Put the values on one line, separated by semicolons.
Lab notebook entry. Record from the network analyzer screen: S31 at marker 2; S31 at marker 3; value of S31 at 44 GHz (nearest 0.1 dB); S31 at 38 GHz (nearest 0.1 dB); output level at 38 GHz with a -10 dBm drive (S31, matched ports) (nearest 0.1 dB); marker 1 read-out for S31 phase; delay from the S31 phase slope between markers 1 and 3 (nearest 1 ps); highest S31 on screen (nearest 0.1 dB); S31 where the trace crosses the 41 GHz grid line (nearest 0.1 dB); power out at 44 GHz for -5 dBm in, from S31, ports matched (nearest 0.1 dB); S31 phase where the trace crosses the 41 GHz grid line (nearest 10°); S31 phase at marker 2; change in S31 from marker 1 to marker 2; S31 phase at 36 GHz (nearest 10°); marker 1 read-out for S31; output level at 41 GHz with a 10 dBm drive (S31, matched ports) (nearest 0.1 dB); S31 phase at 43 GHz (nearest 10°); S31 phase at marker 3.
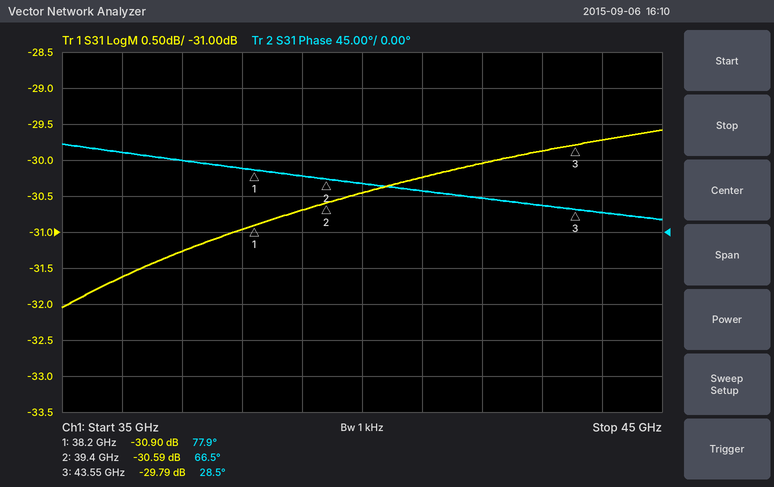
-30.59 dB; -29.79 dB; -29.7 dB; -31.0 dB; -41.0 dBm; 77.9°; 26 ps; -29.6 dB; -30.2 dB; -34.7 dBm; 50°; 66.5°; 0.31 dB; 100°; -30.90 dB; -20.2 dBm; 30°; 28.5°
